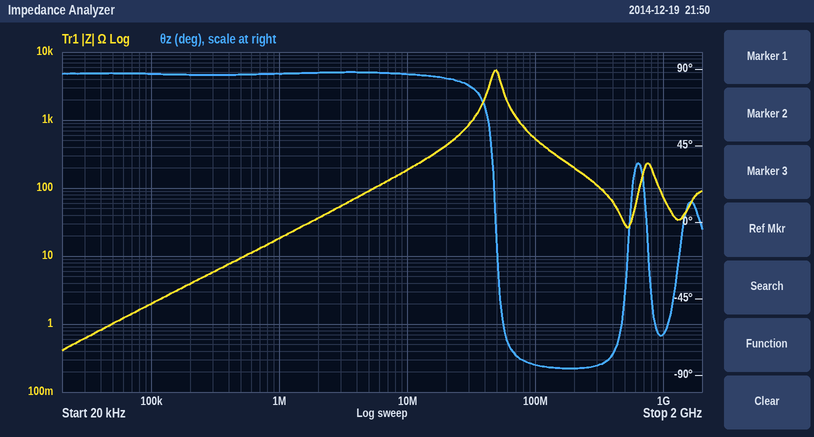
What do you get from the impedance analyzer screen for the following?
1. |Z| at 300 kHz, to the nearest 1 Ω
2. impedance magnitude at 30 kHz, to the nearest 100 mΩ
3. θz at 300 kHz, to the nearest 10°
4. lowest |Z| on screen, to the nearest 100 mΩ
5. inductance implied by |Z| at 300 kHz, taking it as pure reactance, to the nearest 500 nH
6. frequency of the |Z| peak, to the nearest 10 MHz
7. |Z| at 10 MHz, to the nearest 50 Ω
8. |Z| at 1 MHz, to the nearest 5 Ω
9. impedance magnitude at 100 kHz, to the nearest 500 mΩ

6 Ω
600 mΩ
90°
400 mΩ
3.0 µH
50 MHz
200 Ω
20 Ω
2.0 Ω
